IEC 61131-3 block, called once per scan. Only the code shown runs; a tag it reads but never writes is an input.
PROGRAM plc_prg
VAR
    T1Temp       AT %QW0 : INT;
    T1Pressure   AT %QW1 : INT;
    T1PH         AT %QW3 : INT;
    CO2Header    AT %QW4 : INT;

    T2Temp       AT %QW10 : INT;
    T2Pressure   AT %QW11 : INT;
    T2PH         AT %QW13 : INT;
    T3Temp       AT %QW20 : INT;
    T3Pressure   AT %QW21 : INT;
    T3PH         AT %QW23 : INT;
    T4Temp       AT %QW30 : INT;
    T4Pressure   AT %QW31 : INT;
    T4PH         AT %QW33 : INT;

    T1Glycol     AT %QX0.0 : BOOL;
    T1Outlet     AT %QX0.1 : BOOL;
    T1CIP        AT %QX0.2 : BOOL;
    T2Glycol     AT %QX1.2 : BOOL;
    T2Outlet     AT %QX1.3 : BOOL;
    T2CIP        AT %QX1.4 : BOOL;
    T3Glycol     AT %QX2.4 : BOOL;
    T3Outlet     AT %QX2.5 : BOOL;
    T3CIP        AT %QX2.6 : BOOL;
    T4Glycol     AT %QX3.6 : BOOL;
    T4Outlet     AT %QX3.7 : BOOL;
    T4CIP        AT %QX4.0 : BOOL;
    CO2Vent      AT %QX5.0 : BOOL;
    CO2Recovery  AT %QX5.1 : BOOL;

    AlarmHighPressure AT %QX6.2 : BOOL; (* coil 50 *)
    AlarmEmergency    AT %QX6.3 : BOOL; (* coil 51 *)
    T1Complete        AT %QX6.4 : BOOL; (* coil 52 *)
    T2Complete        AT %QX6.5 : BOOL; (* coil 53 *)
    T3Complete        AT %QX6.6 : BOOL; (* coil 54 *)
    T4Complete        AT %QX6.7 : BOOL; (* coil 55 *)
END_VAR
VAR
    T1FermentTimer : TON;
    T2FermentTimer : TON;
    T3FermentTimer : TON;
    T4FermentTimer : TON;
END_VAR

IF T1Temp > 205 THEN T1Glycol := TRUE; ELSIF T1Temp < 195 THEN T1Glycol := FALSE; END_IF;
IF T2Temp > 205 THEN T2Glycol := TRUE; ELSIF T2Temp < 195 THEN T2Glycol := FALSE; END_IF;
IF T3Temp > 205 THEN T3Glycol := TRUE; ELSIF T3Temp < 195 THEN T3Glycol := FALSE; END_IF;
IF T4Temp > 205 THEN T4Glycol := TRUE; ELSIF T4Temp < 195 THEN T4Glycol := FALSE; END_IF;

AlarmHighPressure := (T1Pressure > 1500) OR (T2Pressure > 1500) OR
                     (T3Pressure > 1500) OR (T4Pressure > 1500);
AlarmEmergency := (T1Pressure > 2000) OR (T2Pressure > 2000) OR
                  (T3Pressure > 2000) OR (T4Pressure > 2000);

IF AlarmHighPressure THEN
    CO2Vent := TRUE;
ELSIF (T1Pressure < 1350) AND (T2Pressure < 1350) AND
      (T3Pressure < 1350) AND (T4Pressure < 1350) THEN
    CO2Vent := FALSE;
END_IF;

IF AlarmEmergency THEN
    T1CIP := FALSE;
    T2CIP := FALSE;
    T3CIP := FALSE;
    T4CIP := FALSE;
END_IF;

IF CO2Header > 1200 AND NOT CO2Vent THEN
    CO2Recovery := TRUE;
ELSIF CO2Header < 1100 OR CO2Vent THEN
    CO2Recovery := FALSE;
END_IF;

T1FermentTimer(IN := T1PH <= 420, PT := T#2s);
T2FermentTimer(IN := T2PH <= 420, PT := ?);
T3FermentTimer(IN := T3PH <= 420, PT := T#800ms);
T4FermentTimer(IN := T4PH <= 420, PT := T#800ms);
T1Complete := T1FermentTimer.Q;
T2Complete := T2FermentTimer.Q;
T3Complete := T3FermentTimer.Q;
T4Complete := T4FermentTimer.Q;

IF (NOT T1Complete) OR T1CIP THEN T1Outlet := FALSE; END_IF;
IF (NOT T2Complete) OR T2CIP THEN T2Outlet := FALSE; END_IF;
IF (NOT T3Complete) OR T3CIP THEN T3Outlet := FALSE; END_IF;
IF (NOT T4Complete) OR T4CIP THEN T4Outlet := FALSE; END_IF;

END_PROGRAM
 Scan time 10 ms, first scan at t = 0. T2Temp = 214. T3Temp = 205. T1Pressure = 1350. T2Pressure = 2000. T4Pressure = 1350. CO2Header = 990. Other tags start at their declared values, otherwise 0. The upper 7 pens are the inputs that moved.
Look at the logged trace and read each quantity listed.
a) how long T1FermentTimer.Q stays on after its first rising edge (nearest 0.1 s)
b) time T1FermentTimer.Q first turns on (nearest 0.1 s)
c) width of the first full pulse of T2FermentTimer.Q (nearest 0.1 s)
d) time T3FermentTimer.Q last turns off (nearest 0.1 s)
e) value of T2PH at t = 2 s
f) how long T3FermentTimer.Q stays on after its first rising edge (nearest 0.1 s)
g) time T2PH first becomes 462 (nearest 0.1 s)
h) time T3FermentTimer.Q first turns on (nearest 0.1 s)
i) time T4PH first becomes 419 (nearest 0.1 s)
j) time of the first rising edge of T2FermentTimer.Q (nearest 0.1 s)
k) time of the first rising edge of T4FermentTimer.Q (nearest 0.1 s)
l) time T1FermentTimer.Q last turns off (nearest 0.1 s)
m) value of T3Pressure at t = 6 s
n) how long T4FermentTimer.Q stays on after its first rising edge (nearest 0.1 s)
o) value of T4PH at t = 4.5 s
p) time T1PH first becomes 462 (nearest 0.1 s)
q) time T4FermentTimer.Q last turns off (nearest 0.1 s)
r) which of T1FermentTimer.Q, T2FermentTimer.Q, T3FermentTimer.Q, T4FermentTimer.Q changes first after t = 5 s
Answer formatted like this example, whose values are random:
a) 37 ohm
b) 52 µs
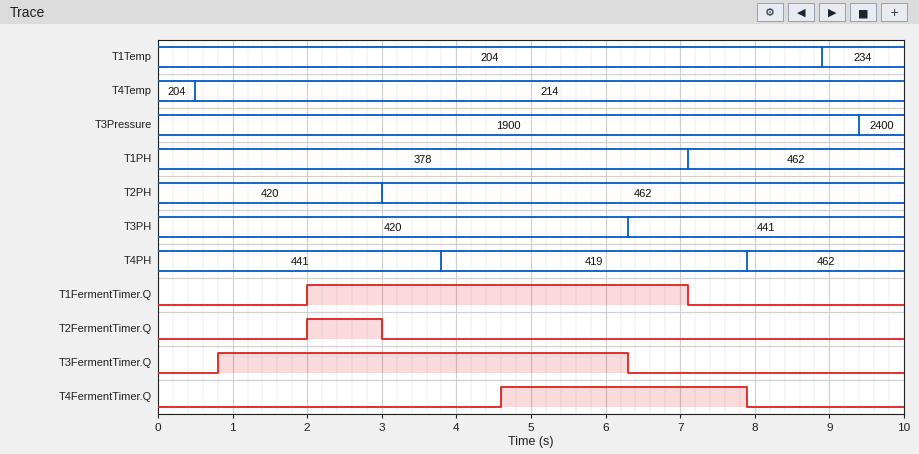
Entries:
a) 5.1 s
b) 2.0 s
c) 1.0 s
d) 6.3 s
e) 420
f) 5.5 s
g) 3.0 s
h) 0.8 s
i) 3.8 s
j) 2.0 s
k) 4.6 s
l) 7.1 s
m) 1900
n) 3.3 s
o) 419
p) 7.1 s
q) 7.9 s
r) T3FermentTimer.Q
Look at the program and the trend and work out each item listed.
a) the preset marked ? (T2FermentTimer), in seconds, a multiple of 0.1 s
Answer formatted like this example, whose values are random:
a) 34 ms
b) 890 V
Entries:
a) 2.0 s
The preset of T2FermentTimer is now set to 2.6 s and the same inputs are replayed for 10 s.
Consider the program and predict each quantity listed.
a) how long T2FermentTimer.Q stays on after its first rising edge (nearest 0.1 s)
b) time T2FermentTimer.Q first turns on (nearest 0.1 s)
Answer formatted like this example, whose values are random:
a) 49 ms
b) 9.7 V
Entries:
a) 0.4 s
b) 2.6 s
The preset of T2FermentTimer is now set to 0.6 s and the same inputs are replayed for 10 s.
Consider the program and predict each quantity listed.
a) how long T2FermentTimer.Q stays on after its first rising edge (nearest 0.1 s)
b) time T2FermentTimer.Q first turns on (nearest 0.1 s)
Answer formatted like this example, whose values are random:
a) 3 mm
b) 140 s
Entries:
a) 2.4 s
b) 0.6 s
